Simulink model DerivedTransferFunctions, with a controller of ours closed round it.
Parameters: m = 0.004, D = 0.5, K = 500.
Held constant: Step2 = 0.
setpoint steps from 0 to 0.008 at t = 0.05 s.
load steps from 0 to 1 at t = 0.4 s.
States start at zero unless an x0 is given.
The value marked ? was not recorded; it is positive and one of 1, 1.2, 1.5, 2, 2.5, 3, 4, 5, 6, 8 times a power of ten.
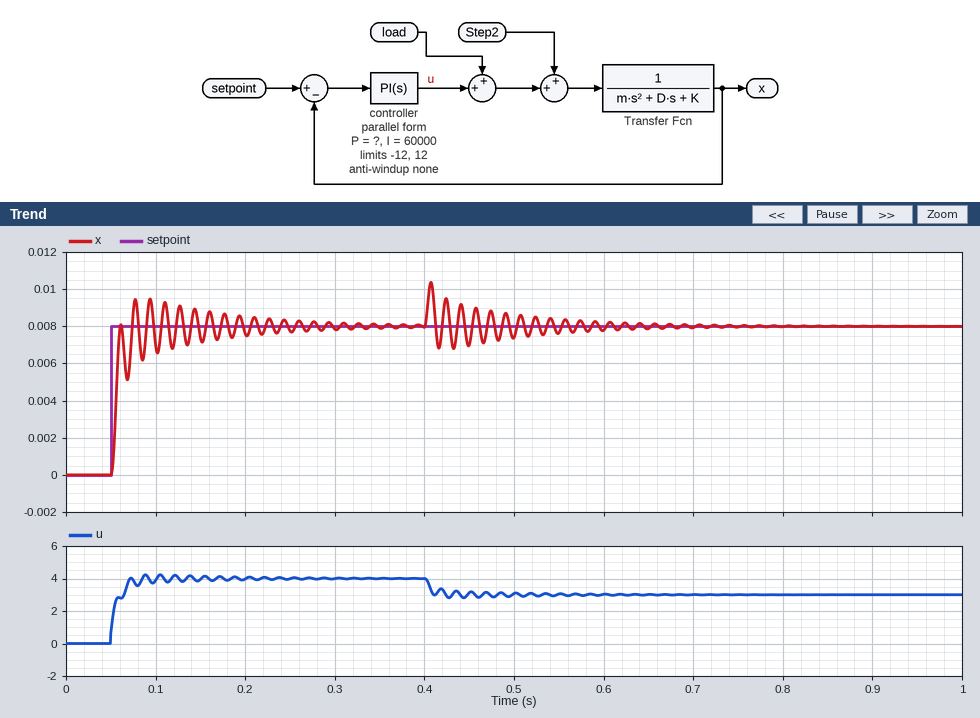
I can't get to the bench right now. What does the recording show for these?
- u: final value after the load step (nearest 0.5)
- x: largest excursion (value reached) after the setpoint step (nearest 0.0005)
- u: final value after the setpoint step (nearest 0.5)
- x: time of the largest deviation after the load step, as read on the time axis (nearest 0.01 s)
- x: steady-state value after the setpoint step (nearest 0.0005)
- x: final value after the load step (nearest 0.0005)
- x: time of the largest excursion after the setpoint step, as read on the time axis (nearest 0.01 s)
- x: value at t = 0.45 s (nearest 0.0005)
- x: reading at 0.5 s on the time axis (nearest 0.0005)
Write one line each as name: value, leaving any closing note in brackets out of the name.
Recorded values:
u: final value after the load step: 3.0
x: largest excursion (value reached) after the setpoint step: 0.0095
u: final value after the setpoint step: 4.0
x: time of the largest deviation after the load step, as read on the time axis: 0.41 s
x: steady-state value after the setpoint step: 0.0080
x: final value after the load step: 0.0080
x: time of the largest excursion after the setpoint step, as read on the time axis: 0.09 s
x: value at t = 0.45 s: 0.0070
x: reading at 0.5 s on the time axis: 0.0075
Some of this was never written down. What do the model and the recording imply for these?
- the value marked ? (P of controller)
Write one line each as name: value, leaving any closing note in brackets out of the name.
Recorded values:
the value marked ?: 80
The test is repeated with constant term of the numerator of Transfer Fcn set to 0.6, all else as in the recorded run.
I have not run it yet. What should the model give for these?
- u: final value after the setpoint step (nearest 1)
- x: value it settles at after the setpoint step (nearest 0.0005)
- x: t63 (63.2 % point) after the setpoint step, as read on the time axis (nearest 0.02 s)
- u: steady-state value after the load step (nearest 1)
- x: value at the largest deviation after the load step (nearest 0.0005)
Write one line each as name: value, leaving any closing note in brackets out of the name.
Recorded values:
u: final value after the setpoint step: 7
x: value it settles at after the setpoint step: 0.0080
x: t63 (63.2 % point) after the setpoint step, as read on the time axis: 0.06 s
u: steady-state value after the load step: 6
x: value at the largest deviation after the load step: 0.0095
